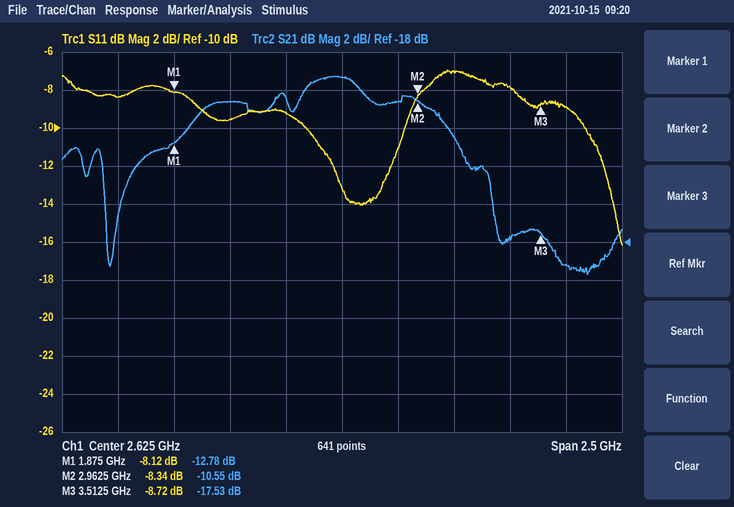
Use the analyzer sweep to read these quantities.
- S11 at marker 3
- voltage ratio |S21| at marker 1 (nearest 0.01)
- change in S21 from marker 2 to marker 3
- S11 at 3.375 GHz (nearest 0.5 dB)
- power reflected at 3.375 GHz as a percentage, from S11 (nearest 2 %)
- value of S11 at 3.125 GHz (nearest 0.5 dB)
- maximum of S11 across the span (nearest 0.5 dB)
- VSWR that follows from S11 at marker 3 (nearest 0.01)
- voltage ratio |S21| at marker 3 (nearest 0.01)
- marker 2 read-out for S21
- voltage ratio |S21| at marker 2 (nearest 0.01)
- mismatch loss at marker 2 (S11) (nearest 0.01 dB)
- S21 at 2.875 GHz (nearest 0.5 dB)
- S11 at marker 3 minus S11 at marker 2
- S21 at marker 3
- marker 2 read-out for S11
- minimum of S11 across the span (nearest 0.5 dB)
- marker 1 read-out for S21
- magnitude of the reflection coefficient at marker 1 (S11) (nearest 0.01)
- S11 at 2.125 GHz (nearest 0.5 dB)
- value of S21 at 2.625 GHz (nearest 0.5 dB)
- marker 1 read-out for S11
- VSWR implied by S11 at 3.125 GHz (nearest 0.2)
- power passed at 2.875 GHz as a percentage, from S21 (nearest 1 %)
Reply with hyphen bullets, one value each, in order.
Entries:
- -8.72 dB
- 0.23
- -6.98 dB
- -8.0 dB
- 16 %
- -7.0 dB
- -7.0 dB
- 2.16
- 0.13
- -10.55 dB
- 0.30
- 0.69 dB
- -10.5 dB
- -0.38 dB
- -17.53 dB
- -8.34 dB
- -16.0 dB
- -12.78 dB
- 0.39
- -9.5 dB
- -9.5 dB
- -8.12 dB
- 2.6
- 9 %
